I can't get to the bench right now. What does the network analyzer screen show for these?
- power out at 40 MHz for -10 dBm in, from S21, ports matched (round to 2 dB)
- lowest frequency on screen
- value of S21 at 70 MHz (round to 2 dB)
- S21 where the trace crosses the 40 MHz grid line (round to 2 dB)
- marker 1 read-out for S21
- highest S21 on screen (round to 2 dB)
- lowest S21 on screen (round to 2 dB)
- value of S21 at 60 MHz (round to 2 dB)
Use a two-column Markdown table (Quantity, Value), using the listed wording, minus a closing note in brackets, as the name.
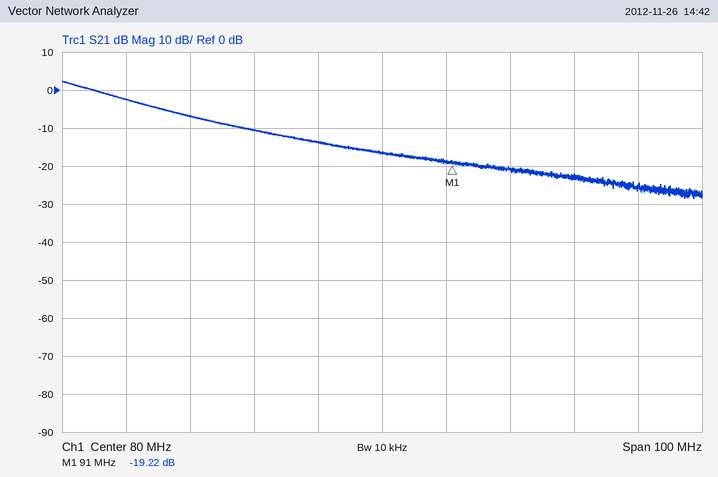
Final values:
| Quantity | Value |
|---|---|
| power out at 40 MHz for -10 dBm in, from S21, ports matched | -12 dBm |
| lowest frequency on screen | 30 MHz |
| value of S21 at 70 MHz | -14 dB |
| S21 where the trace crosses the 40 MHz grid line | -2 dB |
| marker 1 read-out for S21 | -19.22 dB |
| highest S21 on screen | 2 dB |
| lowest S21 on screen | -28 dB |
| value of S21 at 60 MHz | -10 dB |
